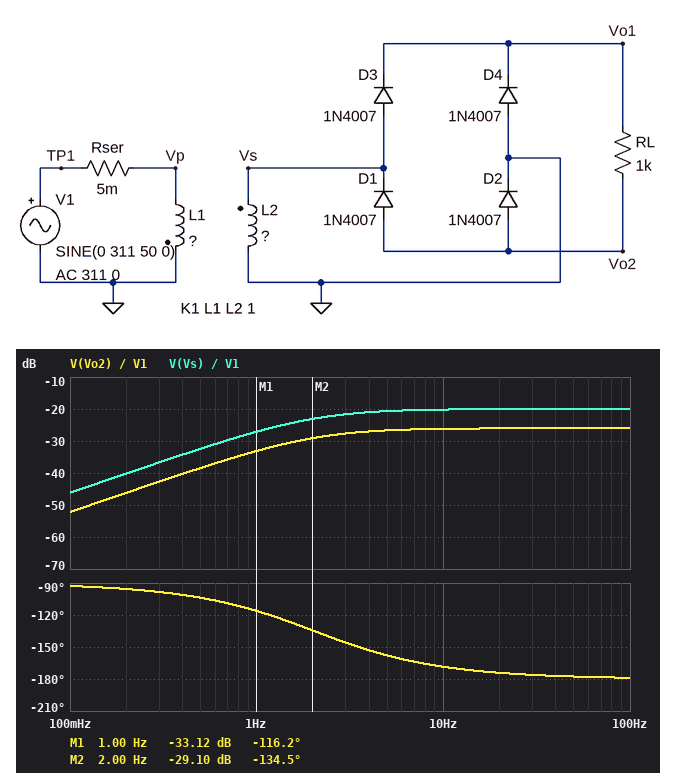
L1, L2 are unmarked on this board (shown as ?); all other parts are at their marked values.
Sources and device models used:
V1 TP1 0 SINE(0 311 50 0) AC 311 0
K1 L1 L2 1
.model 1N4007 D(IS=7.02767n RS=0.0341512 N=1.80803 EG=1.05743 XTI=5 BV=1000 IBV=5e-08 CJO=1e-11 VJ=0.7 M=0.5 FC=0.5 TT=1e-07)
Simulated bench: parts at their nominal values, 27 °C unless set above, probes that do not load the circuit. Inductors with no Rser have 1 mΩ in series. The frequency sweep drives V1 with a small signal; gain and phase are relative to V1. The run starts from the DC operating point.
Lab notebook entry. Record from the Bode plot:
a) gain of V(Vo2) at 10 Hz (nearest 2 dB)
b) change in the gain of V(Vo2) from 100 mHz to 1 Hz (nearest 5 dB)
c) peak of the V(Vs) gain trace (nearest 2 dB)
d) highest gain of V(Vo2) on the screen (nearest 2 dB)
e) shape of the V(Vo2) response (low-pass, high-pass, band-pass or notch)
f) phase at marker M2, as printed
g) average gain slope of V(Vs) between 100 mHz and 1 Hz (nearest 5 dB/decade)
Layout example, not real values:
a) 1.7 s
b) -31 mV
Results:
a) -26 dB
b) 20 dB
c) -20 dB
d) -26 dB
e) high-pass
f) -134.5 deg
g) 20 dB/decade
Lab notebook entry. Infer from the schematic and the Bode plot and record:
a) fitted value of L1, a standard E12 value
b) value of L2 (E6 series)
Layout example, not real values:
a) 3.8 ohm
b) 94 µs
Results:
a) 470 µH
b) 4.7 µH
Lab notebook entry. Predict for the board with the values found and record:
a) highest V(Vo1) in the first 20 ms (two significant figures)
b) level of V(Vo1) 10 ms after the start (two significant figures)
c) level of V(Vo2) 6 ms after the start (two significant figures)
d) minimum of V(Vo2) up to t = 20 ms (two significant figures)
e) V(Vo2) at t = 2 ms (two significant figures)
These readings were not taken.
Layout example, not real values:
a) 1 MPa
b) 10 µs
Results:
a) 31 V
b) 1.8 V
c) -27 V
d) -29 V
e) -17 V
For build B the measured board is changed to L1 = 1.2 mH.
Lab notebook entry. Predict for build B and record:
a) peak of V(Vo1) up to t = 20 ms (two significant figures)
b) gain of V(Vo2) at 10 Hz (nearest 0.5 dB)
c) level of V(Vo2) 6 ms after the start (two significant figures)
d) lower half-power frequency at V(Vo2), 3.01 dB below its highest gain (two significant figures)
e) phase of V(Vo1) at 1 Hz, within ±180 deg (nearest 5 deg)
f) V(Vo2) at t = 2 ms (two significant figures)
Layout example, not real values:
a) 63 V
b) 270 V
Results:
a) 19 V
b) -30.0 dB
c) -17 V
d) 800 mHz
e) -140 deg
f) -11 V
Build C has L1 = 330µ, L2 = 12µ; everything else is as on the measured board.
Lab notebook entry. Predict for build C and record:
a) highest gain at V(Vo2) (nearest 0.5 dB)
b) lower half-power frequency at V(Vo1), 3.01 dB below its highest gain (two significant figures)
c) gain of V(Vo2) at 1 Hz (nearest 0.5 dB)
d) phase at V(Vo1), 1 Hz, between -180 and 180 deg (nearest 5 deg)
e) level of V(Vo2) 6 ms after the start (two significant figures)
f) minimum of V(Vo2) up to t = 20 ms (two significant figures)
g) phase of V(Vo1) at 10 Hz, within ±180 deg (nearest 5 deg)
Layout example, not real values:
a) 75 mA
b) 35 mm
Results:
a) -20.5 dB
b) 2.9 Hz
c) -30.0 dB
d) -110 deg
e) -51 V
f) -55 V
g) -165 deg
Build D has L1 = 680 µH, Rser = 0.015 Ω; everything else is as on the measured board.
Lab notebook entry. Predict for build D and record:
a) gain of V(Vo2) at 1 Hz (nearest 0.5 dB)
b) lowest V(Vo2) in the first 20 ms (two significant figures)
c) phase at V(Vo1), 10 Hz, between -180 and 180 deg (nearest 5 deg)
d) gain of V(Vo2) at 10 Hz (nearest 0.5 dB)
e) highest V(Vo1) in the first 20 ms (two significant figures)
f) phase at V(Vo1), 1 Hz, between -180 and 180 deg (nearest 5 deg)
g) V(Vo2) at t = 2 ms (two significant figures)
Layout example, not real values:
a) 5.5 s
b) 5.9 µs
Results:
a) -39.5 dB
b) -23 V
c) -160 deg
d) -28.0 dB
e) 26 V
f) -105 deg
g) -14 V
